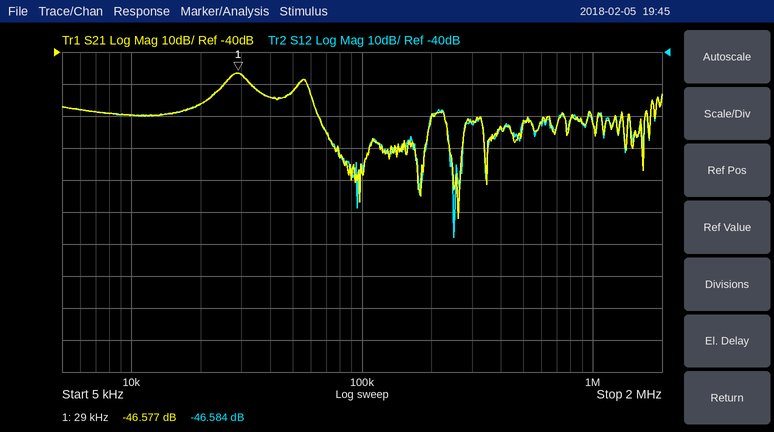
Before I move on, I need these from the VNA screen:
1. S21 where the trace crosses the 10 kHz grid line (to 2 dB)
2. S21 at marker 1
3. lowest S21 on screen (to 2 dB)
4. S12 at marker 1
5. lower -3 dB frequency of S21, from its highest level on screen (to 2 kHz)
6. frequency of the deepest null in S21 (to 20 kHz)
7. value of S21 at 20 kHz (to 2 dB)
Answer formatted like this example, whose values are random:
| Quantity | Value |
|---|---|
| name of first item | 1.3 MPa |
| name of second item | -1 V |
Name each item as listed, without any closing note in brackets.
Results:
| Quantity | Value |
|---|---|
| S21 where the trace crosses the 10 kHz grid line | -60 dB |
| S21 at marker 1 | -46.577 dB |
| lowest S21 on screen | -92 dB |
| S12 at marker 1 | -46.584 dB |
| lower -3 dB frequency of S21, from its highest level on screen | 26 kHz |
| frequency of the deepest null in S21 | 260 kHz |
| value of S21 at 20 kHz | -56 dB |
